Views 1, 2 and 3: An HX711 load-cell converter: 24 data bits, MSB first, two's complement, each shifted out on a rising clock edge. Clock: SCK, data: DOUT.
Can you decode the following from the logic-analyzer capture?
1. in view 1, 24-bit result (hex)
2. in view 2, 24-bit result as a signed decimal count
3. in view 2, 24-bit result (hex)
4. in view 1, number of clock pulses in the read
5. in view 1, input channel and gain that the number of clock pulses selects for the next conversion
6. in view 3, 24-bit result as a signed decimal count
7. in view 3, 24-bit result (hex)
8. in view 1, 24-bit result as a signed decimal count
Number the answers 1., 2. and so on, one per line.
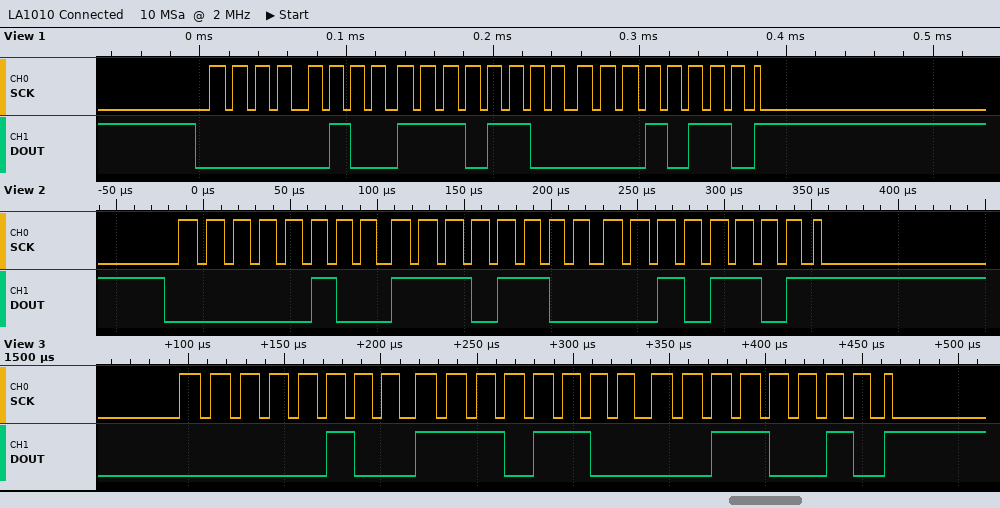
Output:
1. 0x04EC16
2. 322605
3. 0x04EC2D
4. 25
5. channel A, gain 128
6. 322610
7. 0x04EC32
8. 322582
